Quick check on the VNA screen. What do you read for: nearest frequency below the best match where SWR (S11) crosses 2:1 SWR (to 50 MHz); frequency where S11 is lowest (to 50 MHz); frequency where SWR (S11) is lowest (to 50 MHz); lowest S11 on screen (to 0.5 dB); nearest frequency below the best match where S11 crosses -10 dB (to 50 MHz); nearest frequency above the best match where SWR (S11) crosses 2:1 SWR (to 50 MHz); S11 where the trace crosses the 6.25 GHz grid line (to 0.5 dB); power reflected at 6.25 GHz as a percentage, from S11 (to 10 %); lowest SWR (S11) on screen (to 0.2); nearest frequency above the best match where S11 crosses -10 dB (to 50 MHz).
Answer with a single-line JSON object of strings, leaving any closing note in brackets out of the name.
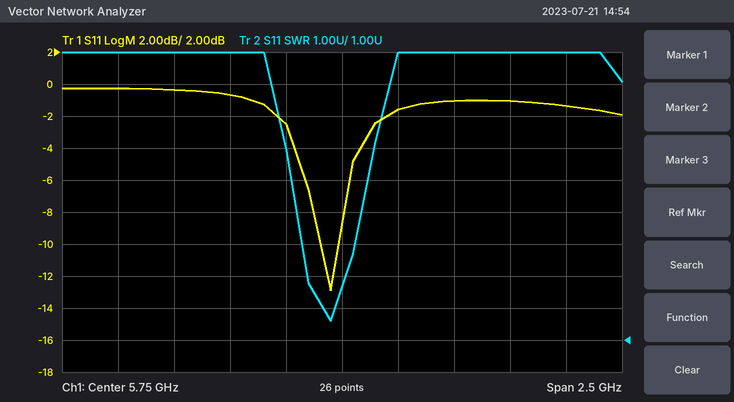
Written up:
{"nearest frequency below the best match where SWR (S11) crosses 2:1 SWR": "5.65 GHz", "frequency where S11 is lowest": "5.70 GHz", "frequency where SWR (S11) is lowest": "5.70 GHz", "lowest S11 on screen": "-13.0 dB", "nearest frequency below the best match where S11 crosses -10 dB": "5.65 GHz", "nearest frequency above the best match where SWR (S11) crosses 2:1 SWR": "5.70 GHz", "S11 where the trace crosses the 6.25 GHz grid line": "-1.0 dB", "power reflected at 6.25 GHz as a percentage, from S11": "80 %", "lowest SWR (S11) on screen": "1.6", "nearest frequency above the best match where S11 crosses -10 dB": "5.75 GHz"}
